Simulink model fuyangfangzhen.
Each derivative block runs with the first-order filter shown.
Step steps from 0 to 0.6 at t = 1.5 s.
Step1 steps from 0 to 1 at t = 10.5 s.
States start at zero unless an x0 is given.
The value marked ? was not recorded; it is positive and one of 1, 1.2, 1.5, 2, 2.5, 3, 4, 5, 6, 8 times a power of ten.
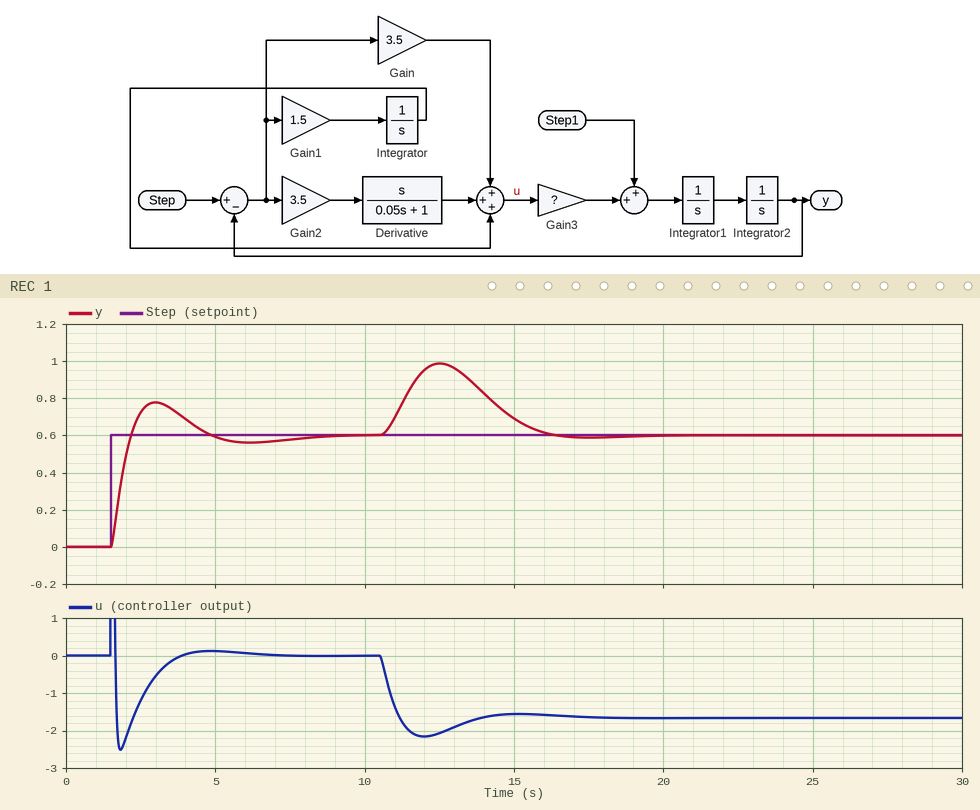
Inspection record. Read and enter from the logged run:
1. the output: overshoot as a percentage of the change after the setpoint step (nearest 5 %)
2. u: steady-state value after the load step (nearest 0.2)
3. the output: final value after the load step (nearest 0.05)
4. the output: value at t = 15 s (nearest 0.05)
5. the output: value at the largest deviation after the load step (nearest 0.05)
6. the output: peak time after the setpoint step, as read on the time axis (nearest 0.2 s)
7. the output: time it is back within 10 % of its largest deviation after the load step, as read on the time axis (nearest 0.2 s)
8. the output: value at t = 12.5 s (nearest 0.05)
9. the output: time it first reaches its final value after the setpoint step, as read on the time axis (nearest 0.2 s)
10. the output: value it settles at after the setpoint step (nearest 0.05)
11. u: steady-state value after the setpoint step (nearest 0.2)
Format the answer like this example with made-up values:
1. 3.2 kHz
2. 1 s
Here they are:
1. 30 %
2. -1.6
3. 0.60
4. 0.70
5. 1.00
6. 3.0 s
7. 15.6 s
8. 1.00
9. 2.2 s
10. 0.60
11. 0.0
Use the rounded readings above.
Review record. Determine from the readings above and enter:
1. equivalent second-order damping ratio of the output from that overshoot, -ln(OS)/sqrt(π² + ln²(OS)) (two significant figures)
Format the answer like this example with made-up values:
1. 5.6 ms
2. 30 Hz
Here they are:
1. 0.36
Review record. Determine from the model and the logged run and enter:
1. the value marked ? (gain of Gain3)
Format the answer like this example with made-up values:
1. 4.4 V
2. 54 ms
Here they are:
1. 0.6
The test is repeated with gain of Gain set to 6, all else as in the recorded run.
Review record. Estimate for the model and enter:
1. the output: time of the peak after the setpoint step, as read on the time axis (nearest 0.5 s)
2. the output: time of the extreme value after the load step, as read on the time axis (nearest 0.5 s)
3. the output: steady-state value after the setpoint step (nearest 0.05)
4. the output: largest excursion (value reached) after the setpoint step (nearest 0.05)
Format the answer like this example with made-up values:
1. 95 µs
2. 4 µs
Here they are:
1. 2.5 s
2. 12.0 s
3. 0.60
4. 0.80
